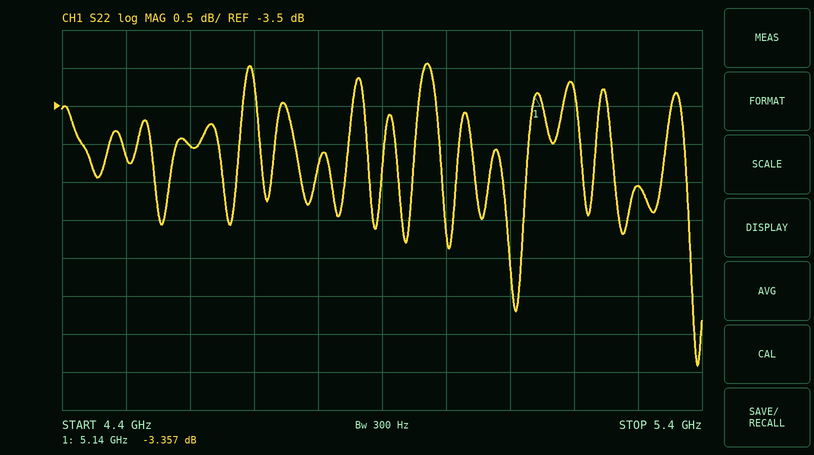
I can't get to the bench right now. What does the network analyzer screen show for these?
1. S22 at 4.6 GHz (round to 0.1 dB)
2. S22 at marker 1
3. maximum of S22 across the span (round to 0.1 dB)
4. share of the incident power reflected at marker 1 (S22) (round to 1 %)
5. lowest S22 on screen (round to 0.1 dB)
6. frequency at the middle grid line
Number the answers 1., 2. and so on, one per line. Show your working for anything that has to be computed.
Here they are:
1. -4.0 dB
2. -3.357 dB
3. -2.9 dB
4. 10^(-3.357/10) ≈ 46 %
5. -6.9 dB
6. 4.9 GHz
